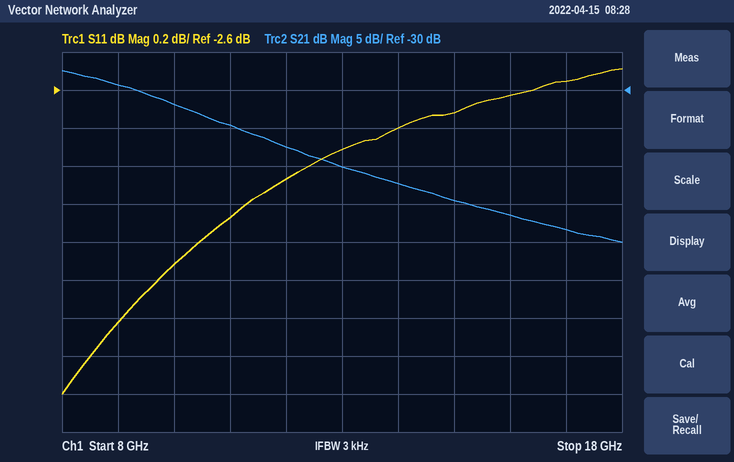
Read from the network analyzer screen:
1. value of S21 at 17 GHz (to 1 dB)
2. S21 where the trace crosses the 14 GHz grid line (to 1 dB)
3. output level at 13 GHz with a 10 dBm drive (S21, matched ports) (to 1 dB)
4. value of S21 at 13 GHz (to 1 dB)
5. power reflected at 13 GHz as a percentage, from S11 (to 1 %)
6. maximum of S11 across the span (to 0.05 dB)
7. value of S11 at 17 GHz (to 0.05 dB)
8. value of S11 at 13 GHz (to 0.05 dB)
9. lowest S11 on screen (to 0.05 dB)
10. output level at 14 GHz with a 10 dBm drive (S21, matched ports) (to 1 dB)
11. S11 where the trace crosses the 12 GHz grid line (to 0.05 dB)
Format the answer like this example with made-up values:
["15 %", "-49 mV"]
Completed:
["-48 dB", "-42 dB", "-30 dBm", "-40 dB", "51 %", "-2.50 dB", "-2.55 dB", "-2.90 dB", "-4.20 dB", "-32 dBm", "-3.05 dB"]
